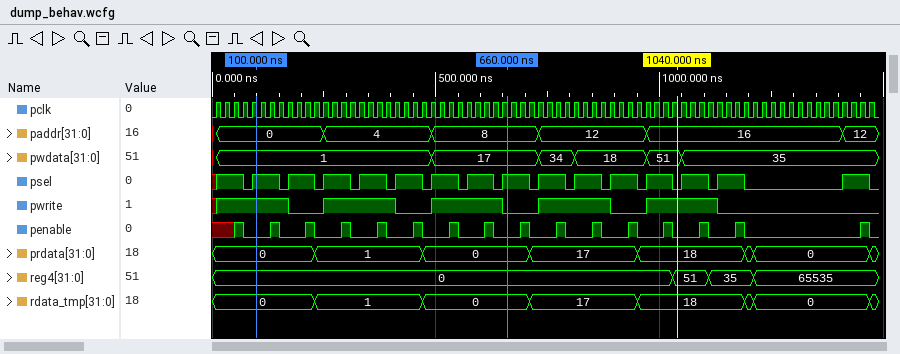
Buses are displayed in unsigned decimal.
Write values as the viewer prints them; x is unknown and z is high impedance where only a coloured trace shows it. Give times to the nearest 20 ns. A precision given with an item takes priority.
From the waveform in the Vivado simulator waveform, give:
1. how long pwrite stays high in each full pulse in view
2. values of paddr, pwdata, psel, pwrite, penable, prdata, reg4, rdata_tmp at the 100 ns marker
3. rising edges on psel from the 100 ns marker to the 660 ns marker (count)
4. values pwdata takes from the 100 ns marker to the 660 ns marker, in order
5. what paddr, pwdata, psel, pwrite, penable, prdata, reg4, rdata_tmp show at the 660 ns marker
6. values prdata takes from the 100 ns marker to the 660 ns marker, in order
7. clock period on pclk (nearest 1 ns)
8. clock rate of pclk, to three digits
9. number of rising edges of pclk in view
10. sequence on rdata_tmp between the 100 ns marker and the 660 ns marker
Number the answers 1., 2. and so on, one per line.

1. 160 ns, 160 ns, 160 ns, 160 ns
2. paddr=0, pwdata=1, psel=1, pwrite=1, penable=0, prdata=0, reg4=0, rdata_tmp=0
3. 7
4. 1, 17
5. paddr=8, pwdata=17, psel=1, pwrite=0, penable=0, prdata=0, reg4=0, rdata_tmp=0
6. 0, 1, 0
7. 20 ns
8. 50.0 MHz
9. 74
10. 0, 1, 0
